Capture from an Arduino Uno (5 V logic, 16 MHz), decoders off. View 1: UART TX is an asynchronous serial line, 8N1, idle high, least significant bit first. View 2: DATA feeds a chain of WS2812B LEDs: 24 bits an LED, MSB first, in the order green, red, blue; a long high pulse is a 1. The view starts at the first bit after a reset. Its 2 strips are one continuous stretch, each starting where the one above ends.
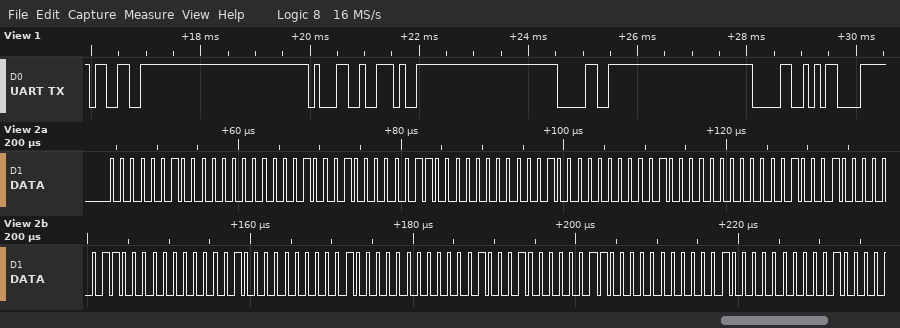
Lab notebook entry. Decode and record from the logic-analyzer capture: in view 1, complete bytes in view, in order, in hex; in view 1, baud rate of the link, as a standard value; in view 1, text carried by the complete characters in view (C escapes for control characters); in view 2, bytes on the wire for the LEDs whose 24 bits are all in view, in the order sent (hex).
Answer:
33 31 2E 30 30 0D
9600 baud
"31.00\r"
02 00 11 03 00 10 02 00 11 03 00 10 02 00 11 03 00 10
